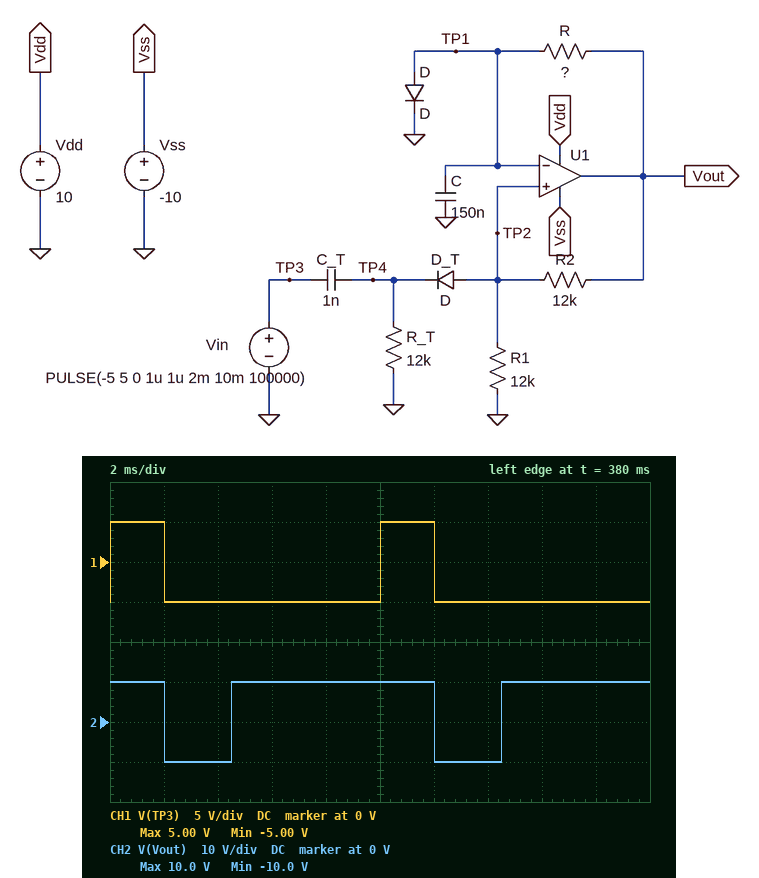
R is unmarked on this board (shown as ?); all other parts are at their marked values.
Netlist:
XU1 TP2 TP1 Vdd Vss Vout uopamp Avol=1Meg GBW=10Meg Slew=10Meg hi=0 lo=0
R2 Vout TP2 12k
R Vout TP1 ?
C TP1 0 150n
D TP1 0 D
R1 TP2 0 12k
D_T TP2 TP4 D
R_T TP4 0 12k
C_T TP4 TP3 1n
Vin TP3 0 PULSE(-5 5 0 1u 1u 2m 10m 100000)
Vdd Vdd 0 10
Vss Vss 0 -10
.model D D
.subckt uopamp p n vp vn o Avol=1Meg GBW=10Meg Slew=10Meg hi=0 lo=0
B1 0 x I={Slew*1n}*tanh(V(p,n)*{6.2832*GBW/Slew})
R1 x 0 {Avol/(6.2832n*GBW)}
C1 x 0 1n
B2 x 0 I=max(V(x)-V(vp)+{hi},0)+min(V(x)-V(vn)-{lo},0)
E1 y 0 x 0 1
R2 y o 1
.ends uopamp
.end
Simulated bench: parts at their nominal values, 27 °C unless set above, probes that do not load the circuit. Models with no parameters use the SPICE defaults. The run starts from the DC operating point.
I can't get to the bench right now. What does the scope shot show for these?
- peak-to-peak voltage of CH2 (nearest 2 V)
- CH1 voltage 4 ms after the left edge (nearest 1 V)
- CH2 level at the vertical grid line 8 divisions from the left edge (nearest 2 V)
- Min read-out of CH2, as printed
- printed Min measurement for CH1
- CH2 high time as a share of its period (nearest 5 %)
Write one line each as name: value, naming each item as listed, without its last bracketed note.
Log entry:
peak-to-peak voltage of CH2: 20 V
CH1 voltage 4 ms after the left edge: -5 V
CH2 level at the vertical grid line 8 divisions from the left edge: 10 V
Min read-out of CH2, as printed: -10.0 V
printed Min measurement for CH1: -5.00 V
CH2 high time as a share of its period: 75 %
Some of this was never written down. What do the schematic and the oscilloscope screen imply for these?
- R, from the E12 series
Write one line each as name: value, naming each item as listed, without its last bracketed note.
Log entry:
R, from the E12 series: 22 kΩ
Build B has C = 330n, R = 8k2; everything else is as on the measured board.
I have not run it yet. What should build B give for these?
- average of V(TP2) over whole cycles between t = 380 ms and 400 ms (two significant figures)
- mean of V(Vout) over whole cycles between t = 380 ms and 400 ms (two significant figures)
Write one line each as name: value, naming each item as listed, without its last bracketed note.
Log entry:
average of V(TP2) over whole cycles between t = 380 ms and 400 ms: 1.8 V
mean of V(Vout) over whole cycles between t = 380 ms and 400 ms: 5.9 V
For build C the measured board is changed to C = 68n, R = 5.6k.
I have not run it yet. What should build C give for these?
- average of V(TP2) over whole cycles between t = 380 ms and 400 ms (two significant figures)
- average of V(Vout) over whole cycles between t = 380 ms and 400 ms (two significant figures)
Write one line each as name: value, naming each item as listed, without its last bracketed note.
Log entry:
average of V(TP2) over whole cycles between t = 380 ms and 400 ms: 3.3 V
average of V(Vout) over whole cycles between t = 380 ms and 400 ms: 9.4 V
